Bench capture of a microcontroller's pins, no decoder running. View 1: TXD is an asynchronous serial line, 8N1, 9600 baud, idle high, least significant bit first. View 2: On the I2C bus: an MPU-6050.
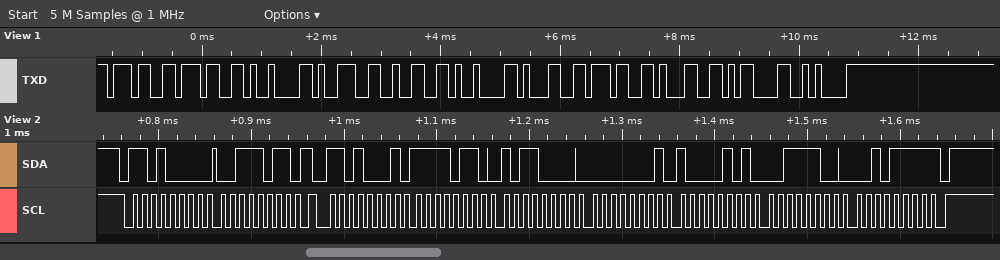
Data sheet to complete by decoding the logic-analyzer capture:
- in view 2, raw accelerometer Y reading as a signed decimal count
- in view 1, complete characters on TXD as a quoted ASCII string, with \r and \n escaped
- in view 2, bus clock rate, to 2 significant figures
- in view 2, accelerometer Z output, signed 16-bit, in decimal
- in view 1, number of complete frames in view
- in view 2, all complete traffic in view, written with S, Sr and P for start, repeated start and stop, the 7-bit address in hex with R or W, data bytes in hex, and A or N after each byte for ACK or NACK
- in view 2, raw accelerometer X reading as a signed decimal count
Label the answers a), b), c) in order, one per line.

a) 389
b) "77\t92\t171\r\n"
c) 100 kHz
d) 15407
e) 11
f) S 68W A 3B A Sr 68R A F6 A B0 A 01 A 85 A 3C A 2F N P
g) -2384
